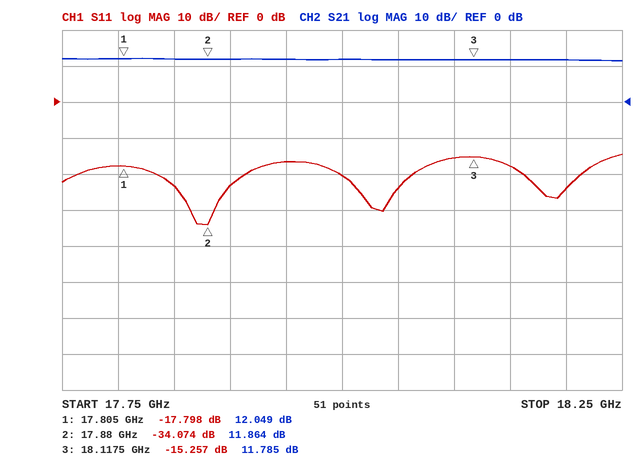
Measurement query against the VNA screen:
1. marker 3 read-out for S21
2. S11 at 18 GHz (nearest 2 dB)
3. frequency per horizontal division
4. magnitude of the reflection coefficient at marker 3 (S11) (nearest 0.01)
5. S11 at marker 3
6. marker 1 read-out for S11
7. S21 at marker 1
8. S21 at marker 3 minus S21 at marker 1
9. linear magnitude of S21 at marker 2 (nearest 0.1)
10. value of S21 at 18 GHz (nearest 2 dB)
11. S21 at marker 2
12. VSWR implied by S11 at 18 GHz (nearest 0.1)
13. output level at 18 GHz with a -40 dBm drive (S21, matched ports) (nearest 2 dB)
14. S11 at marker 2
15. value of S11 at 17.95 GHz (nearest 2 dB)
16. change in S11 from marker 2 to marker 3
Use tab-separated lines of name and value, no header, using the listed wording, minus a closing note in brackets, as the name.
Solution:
marker 3 read-out for S21	11.785 dB
S11 at 18 GHz	-20 dB
frequency per horizontal division	50 MHz
magnitude of the reflection coefficient at marker 3 (S11)	0.17
S11 at marker 3	-15.257 dB
marker 1 read-out for S11	-17.798 dB
S21 at marker 1	12.049 dB
S21 at marker 3 minus S21 at marker 1	-0.264 dB
linear magnitude of S21 at marker 2	3.9
value of S21 at 18 GHz	12 dB
S21 at marker 2	11.864 dB
VSWR implied by S11 at 18 GHz	1.2
output level at 18 GHz with a -40 dBm drive (S21, matched ports)	-28 dBm
S11 at marker 2	-34.074 dB
value of S11 at 17.95 GHz	-16 dB
change in S11 from marker 2 to marker 3	18.817 dB
